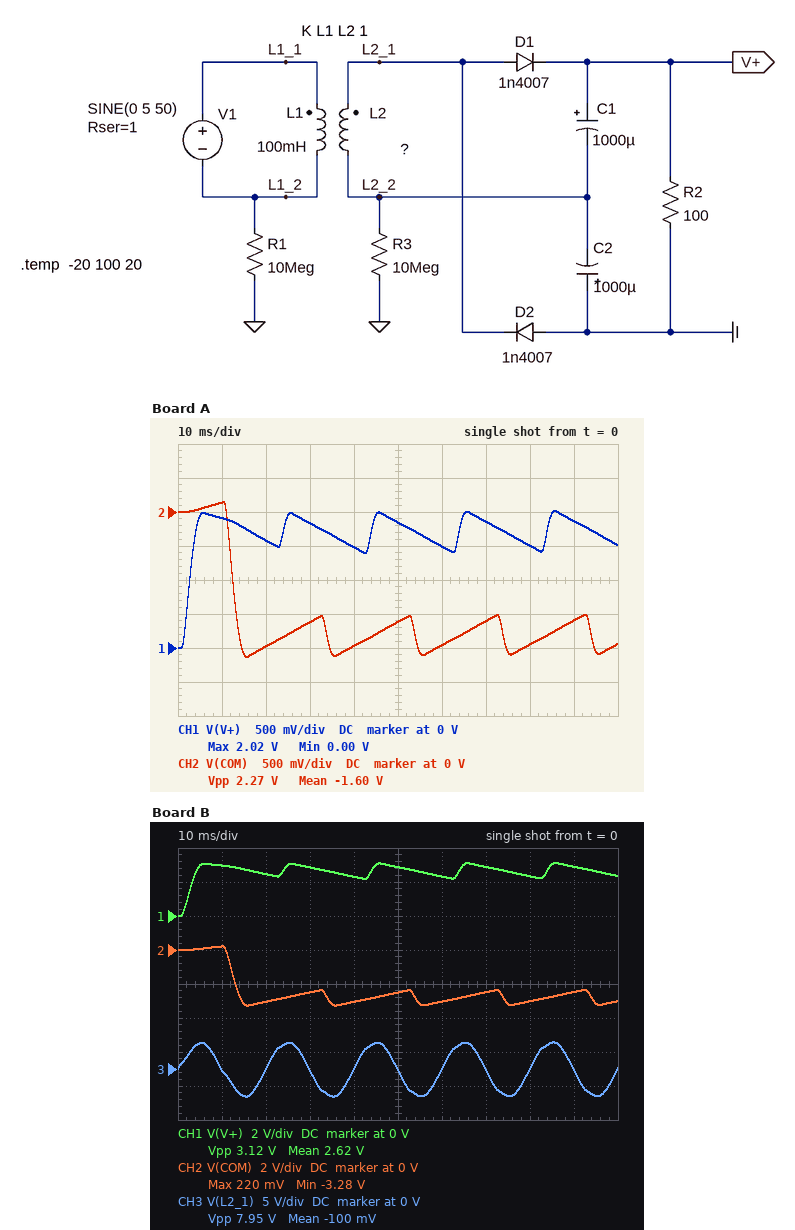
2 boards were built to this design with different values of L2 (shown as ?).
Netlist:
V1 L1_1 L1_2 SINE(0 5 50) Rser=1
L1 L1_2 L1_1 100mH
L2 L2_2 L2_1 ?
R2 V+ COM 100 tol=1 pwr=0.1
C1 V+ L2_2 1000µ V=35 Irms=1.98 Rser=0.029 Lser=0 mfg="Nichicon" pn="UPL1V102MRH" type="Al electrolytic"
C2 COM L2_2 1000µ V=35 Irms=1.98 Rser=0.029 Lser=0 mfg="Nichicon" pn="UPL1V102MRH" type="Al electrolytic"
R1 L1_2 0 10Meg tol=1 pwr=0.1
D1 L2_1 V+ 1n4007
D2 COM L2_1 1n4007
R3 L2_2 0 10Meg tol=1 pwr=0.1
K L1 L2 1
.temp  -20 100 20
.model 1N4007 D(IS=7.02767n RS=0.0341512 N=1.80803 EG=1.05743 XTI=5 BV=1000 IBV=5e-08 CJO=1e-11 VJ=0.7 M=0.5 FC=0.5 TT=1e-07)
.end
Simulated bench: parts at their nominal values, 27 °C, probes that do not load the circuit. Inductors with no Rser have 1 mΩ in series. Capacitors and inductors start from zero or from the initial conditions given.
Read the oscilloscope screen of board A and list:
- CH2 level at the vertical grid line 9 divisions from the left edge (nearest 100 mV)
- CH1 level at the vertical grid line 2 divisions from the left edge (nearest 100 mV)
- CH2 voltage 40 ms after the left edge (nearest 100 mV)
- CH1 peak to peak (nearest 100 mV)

-1.6 V
1.6 V
-2.0 V
2.0 V
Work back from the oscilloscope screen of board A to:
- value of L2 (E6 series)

33 mH
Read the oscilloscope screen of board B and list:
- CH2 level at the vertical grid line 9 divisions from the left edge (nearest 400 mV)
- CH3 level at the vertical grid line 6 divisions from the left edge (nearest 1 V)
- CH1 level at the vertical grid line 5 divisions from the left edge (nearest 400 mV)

-2.4 V
0 V
2.8 V
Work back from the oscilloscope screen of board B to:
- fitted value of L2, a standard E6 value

68 mH
